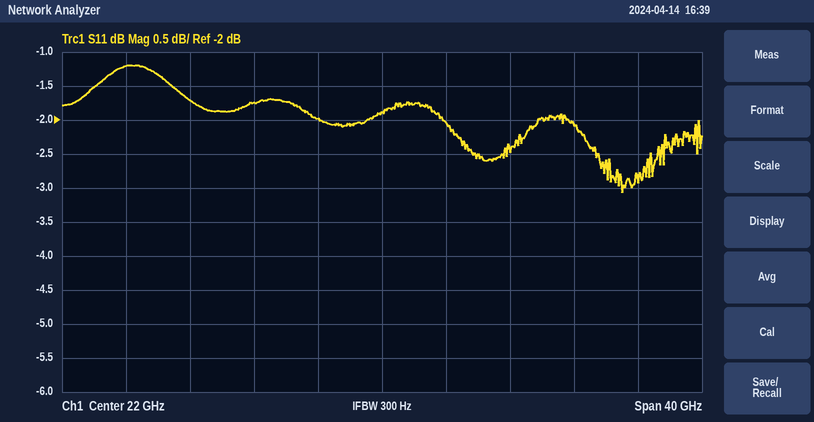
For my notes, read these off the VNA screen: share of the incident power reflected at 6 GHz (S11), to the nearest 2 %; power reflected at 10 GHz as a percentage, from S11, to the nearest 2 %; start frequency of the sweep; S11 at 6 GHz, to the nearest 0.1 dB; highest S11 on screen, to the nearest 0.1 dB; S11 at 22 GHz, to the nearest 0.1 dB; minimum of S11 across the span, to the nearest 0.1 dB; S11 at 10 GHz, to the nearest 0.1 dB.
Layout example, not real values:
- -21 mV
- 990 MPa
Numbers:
- 76 %
- 68 %
- 2 GHz
- -1.2 dB
- -1.2 dB
- -1.9 dB
- -3.1 dB
- -1.7 dB
